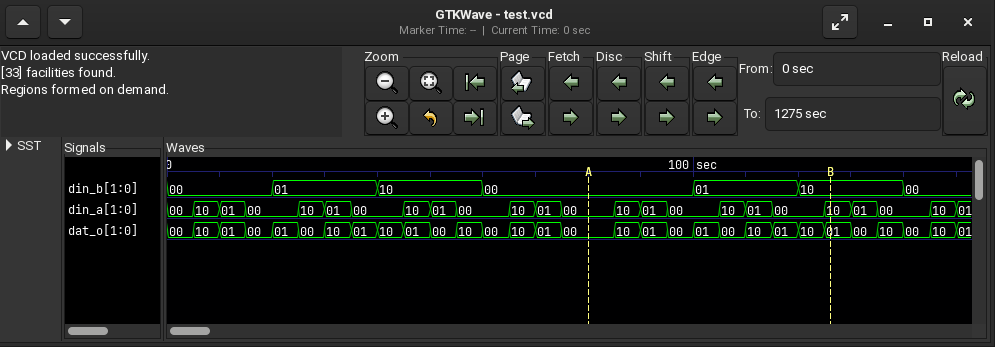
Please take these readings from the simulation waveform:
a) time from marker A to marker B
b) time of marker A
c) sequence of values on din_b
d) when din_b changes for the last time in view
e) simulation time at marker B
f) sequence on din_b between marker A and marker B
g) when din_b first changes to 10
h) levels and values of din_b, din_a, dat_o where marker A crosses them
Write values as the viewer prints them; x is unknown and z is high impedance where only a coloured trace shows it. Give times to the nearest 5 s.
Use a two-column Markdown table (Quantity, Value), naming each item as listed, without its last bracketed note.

| Quantity | Value |
|---|---|
| time from marker A to marker B | 45 s |
| time of marker A | 80 s |
| sequence of values on din_b | 00, 01, 10, 00, 01, 10, 00 |
| when din_b changes for the last time in view | 140 s |
| simulation time at marker B | 125 s |
| sequence on din_b between marker A and marker B | 00, 01, 10 |
| when din_b first changes to 10 | 40 s |
| levels and values of din_b, din_a, dat_o where marker A crosses them | din_b=00, din_a=00, dat_o=00 |
